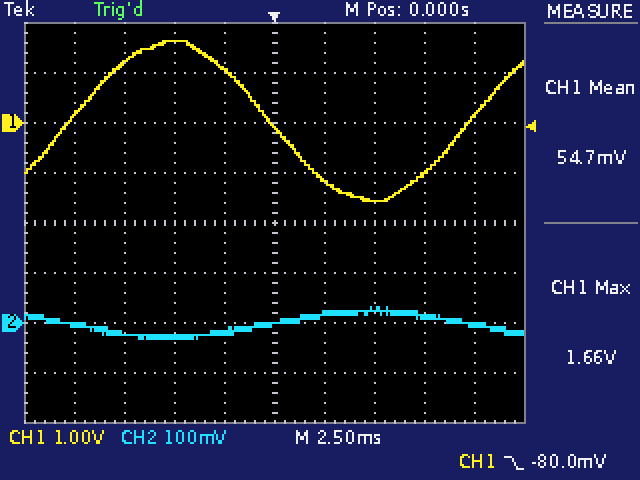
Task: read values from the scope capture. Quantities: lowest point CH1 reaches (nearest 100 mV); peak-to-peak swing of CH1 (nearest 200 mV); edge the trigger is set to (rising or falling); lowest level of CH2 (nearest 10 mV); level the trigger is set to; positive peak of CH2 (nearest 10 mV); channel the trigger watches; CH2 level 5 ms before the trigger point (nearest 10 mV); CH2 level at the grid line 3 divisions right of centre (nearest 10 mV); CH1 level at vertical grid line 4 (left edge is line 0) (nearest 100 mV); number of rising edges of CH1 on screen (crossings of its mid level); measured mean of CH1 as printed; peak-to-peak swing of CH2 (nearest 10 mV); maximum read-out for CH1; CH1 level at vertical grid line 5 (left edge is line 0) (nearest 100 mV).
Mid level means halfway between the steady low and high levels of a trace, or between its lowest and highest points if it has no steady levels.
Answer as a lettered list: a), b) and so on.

a) -1.6 V
b) 3.2 V
c) falling
d) -30 mV
e) -80.0 mV
f) 30 mV
g) CH1
h) -30 mV
i) 10 mV
j) 1.1 V
k) 2
l) 54.7 mV
m) 60 mV
n) 1.66 V
o) -100 mV
